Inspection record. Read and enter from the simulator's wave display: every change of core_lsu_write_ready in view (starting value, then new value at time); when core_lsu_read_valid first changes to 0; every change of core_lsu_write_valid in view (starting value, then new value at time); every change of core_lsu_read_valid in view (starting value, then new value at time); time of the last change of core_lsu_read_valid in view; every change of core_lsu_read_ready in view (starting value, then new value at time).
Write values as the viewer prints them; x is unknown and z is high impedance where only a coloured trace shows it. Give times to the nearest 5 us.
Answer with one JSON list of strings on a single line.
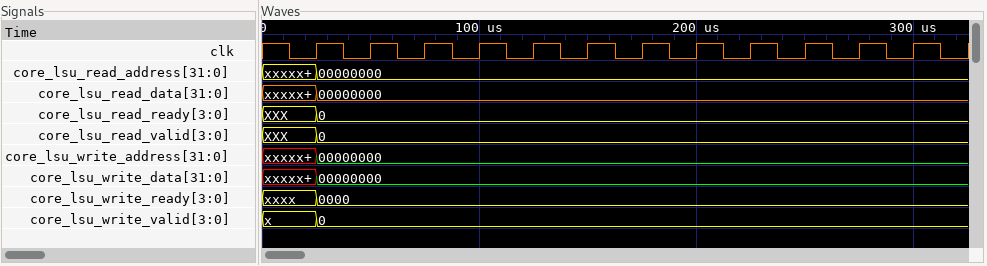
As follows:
["xxxx, 0000 at 25 us", "25 us", "x, 0 at 25 us", "XXX, 0 at 25 us", "25 us", "XXX, 0 at 25 us"]
